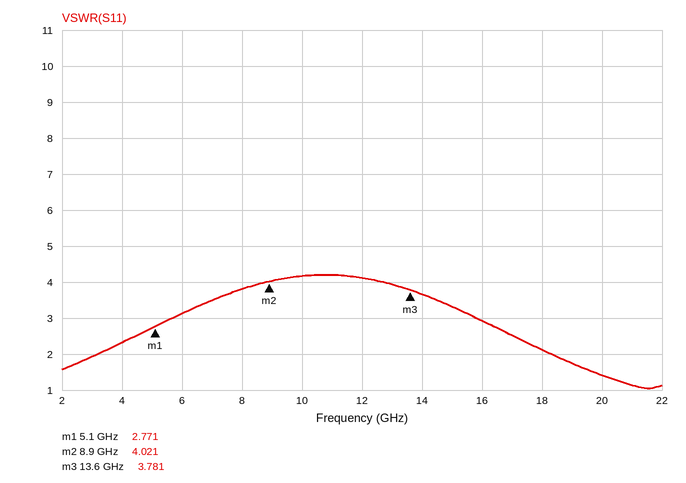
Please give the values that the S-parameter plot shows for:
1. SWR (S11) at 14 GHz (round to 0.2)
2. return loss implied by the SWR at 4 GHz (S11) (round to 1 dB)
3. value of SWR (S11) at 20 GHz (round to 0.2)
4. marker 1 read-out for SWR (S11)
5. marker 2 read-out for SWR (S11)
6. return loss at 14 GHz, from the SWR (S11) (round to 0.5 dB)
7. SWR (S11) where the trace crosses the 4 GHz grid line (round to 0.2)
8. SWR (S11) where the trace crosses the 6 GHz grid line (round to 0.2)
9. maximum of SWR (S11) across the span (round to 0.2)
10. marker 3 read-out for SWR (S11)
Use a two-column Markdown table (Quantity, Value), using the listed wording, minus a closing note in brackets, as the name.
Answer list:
| Quantity | Value |
|---|---|
| SWR (S11) at 14 GHz | 3.6 |
| return loss implied by the SWR at 4 GHz (S11) | 8 dB |
| value of SWR (S11) at 20 GHz | 1.4 |
| marker 1 read-out for SWR | 2.771 |
| marker 2 read-out for SWR | 4.021 |
| return loss at 14 GHz, from the SWR (S11) | 5.0 dB |
| SWR (S11) where the trace crosses the 4 GHz grid line | 2.4 |
| SWR (S11) where the trace crosses the 6 GHz grid line | 3.2 |
| maximum of SWR (S11) across the span | 4.2 |
| marker 3 read-out for SWR | 3.781 |
